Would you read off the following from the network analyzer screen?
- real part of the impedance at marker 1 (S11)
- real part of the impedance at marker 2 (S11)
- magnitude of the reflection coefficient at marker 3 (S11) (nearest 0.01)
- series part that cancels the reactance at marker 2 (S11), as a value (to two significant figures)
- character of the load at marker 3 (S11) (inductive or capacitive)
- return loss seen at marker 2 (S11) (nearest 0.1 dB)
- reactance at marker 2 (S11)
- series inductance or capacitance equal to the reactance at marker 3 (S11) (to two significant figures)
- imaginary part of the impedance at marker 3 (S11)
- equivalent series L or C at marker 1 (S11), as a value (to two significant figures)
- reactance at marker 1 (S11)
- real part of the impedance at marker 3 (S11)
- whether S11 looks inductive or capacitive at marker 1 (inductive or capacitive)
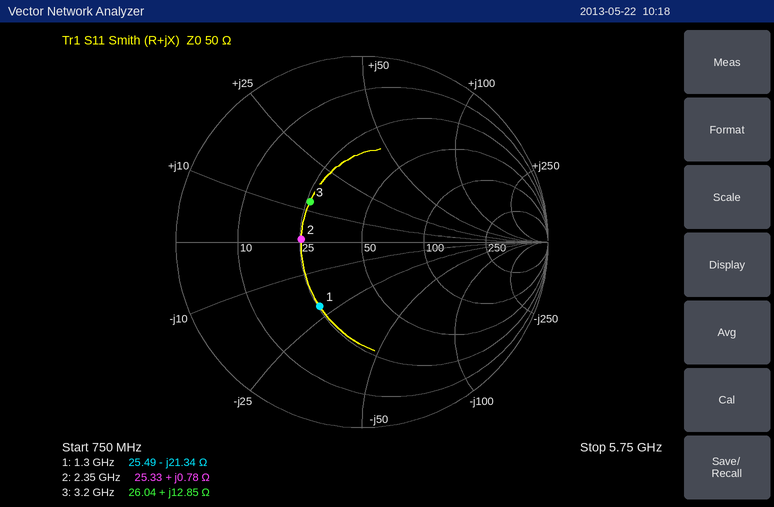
25.49 Ω
25.33 Ω
0.35
87 pF
inductive
9.7 dB
+0.78 Ω
640 pH
+12.85 Ω
5.7 pF
-21.34 Ω
26.04 Ω
capacitive
